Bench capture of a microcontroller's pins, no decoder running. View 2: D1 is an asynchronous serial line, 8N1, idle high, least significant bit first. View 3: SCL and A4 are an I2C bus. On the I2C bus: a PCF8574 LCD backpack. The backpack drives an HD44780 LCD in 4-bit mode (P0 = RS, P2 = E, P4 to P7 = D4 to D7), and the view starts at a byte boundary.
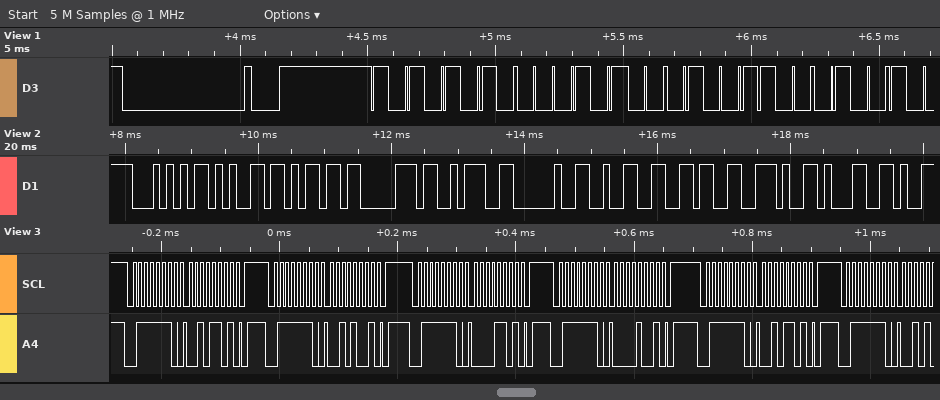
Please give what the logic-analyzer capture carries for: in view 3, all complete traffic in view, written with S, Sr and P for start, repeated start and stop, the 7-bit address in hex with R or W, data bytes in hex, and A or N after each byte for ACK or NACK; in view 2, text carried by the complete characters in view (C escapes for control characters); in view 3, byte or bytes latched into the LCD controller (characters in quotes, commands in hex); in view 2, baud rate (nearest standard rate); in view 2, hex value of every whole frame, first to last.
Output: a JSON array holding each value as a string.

["S 3FW A 2D A P S 3FW A 29 A P S 3FW A 0D A P S 3FW A 09 A P S 3FW A 2D A P S 3FW A", "\"Temp: 26.1\"", "' '", "9600 baud", "54 65 6D 70 3A 20 32 36 2E 31"]
